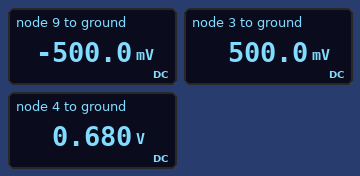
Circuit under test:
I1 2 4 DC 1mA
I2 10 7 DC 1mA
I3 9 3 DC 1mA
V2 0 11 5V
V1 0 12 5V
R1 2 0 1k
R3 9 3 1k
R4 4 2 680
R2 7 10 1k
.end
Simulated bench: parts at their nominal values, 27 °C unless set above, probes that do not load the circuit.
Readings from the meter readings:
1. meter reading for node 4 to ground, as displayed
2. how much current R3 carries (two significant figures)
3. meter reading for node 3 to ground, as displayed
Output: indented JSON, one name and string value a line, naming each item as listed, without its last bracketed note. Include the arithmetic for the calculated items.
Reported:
{
  "meter reading for node 4 to ground, as displayed": "0.680 V",
  "how much current R3 carries": "(500 mV - (-500 mV)) / 1 kΩ = 1.0 mA",
  "meter reading for node 3 to ground, as displayed": "500.0 mV"
}
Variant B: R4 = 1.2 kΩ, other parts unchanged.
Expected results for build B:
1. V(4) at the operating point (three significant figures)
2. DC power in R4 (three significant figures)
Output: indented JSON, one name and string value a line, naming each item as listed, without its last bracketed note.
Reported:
{
  "V(4) at the operating point": "1.20 V",
  "DC power in R4": "1.20 mW"
}
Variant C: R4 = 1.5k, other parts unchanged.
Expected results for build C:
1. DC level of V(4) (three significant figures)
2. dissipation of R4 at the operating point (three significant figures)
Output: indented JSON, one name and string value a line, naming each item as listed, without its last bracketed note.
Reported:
{
  "DC level of V(4)": "1.50 V",
  "dissipation of R4 at the operating point": "1.50 mW"
}
